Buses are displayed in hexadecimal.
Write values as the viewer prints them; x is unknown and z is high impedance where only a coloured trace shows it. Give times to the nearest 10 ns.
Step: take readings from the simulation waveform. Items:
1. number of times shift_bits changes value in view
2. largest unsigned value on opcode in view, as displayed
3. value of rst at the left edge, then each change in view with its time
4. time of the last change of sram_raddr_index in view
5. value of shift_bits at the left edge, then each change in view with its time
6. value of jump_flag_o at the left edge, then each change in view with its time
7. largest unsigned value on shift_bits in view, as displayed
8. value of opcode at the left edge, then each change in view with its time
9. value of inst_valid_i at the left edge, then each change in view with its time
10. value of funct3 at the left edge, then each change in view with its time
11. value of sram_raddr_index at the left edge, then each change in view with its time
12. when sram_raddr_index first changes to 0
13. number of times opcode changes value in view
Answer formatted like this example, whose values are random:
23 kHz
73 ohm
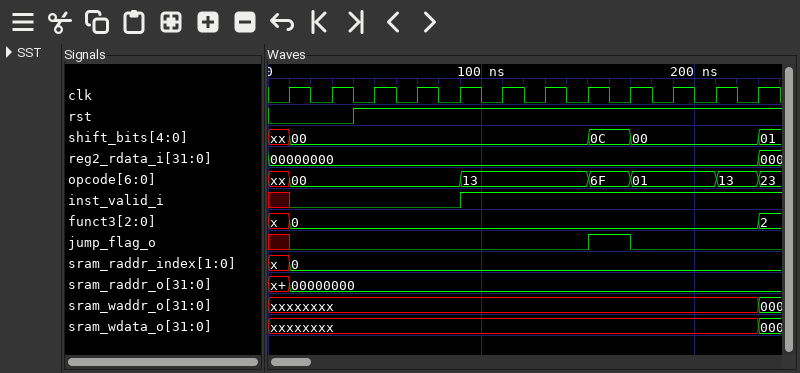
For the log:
4
6F
0, 1 at 40 ns
10 ns
xx, 00 at 10 ns, 0C at 150 ns, 00 at 170 ns, 01 at 230 ns
x, 0 at 10 ns, 1 at 150 ns, 0 at 170 ns
0C
xx, 00 at 10 ns, 13 at 90 ns, 6F at 150 ns, 01 at 170 ns, 13 at 210 ns, 23 at 230 ns
x, 0 at 10 ns, 1 at 90 ns
x, 0 at 10 ns, 2 at 230 ns
x, 0 at 10 ns
10 ns
6
